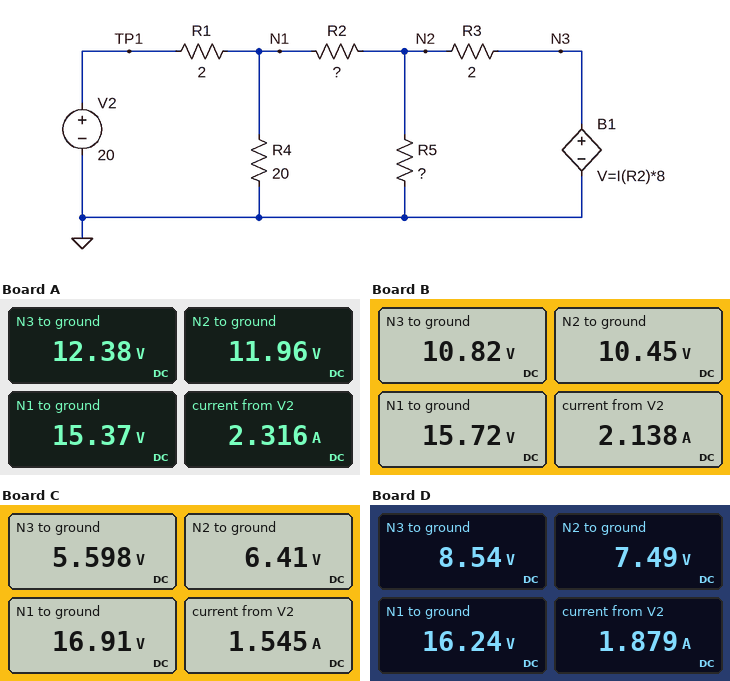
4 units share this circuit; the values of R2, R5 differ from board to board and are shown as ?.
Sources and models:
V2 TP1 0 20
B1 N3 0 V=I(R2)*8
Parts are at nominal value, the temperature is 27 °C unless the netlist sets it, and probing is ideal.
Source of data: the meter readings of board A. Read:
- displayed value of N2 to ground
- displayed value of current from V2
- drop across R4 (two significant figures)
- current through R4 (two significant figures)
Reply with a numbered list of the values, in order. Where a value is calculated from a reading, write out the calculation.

1. 11.96 V
2. 2.316 A
3. 15.37 V = 15 V
4. (15.37 V) / 20 Ω = 770 mA
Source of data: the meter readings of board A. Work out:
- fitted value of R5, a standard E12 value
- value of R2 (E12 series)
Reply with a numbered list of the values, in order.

1. 6.8 Ω
2. 2.2 Ω
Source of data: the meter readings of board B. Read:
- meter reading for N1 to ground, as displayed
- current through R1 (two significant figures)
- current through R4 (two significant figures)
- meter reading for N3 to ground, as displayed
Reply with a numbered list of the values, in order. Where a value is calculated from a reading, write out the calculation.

1. 15.72 V
2. (20 V - 15.72 V) / 2 Ω = 2.1 A
3. (15.72 V) / 20 Ω = 790 mA
4. 10.82 V
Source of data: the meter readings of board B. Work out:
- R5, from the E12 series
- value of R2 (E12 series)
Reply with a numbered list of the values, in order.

1. 6.8 Ω
2. 3.9 Ω
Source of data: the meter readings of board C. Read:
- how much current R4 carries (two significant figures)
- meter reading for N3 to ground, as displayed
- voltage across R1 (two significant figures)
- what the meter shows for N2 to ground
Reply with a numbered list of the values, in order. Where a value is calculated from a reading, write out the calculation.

1. (16.91 V) / 20 Ω = 850 mA
2. 5.598 V
3. 20 V - 16.91 V = 3.1 V
4. 6.41 V
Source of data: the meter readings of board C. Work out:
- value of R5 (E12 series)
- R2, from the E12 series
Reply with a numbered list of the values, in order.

1. 22 Ω
2. 15 Ω
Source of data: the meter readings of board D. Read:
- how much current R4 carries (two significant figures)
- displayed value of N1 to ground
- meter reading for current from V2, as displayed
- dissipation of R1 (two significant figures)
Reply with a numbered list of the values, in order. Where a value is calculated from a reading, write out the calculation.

1. (16.24 V) / 20 Ω = 810 mA
2. 16.24 V
3. 1.879 A
4. (20 V - 16.24 V)^2 / 2 Ω = 7.1 W
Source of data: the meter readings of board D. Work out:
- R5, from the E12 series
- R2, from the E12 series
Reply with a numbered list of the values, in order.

1. 4.7 Ω
2. 8.2 Ω
